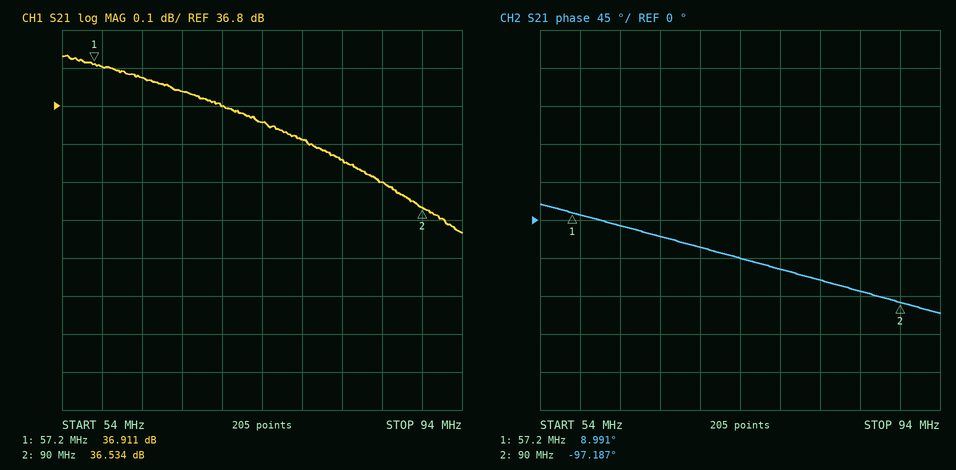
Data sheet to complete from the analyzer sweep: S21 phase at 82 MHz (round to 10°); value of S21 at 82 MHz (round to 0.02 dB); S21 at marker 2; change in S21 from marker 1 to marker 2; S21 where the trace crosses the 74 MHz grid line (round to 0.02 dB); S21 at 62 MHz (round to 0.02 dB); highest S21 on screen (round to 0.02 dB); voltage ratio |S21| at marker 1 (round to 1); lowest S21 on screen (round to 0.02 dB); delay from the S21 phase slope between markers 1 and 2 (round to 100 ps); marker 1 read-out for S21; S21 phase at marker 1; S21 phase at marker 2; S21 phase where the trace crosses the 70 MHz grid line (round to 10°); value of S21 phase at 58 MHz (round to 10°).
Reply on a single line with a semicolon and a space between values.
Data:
-70°; 36.66 dB; 36.534 dB; -0.377 dB; 36.76 dB; 36.88 dB; 36.94 dB; 70; 36.46 dB; 9.0 ns; 36.911 dB; 8.991°; -97.187°; -30°; 10°
